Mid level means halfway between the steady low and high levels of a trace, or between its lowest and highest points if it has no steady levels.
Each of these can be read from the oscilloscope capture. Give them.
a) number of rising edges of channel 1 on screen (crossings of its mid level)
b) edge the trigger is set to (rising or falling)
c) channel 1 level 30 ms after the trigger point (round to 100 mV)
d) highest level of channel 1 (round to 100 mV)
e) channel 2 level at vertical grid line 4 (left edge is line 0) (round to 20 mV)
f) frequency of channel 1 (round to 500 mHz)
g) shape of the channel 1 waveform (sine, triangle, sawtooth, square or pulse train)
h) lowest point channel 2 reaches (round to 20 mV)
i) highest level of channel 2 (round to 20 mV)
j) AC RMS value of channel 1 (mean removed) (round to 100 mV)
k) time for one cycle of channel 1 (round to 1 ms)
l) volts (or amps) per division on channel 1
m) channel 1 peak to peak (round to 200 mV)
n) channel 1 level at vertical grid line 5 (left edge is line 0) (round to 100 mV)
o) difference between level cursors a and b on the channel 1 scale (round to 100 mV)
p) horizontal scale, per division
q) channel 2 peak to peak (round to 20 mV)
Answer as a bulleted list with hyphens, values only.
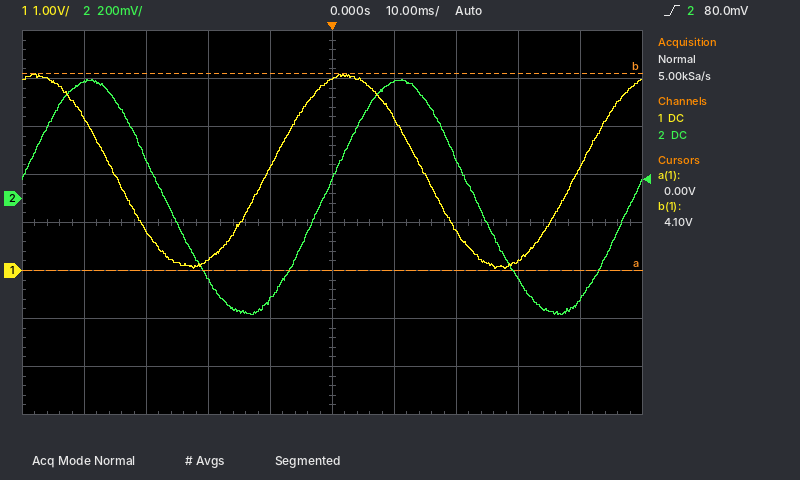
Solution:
- 2
- rising
- 200 mV
- 4.1 V
- -420 mV
- 20.0 Hz
- sine
- -480 mV
- 500 mV
- 1.4 V
- 50 ms
- 1 V
- 4.0 V
- 4.0 V
- 4.1 V
- 10 ms
- 980 mV
